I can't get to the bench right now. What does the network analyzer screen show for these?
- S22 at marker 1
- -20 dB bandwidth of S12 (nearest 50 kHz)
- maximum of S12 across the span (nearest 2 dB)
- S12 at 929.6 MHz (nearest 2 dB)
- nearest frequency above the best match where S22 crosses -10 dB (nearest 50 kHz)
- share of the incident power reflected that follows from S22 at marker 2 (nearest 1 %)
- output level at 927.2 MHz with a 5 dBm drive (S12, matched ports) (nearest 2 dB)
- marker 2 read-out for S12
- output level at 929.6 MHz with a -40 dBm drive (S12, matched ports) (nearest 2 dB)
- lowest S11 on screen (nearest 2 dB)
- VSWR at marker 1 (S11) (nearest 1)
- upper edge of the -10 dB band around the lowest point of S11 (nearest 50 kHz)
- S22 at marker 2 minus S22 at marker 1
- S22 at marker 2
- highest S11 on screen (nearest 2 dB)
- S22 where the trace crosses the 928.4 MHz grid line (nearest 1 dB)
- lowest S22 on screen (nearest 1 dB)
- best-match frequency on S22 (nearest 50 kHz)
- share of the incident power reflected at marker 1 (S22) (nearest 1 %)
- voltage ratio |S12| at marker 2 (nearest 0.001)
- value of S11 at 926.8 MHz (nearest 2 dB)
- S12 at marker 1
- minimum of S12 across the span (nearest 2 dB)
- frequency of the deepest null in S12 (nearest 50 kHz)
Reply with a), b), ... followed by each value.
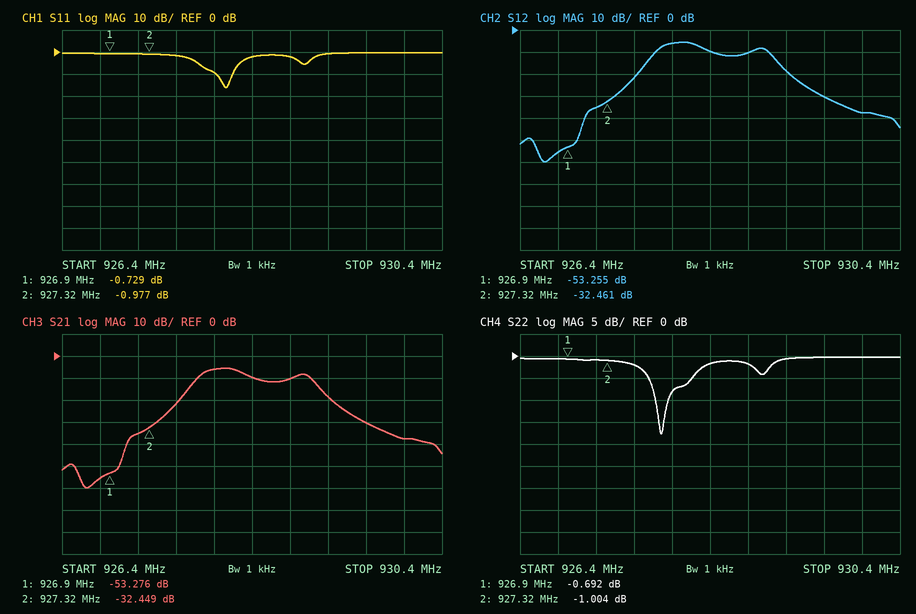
a) -0.692 dB
b) 1.90 MHz
c) -6 dB
d) -30 dB
e) 927.95 MHz
f) 79 %
g) -30 dBm
h) -32.461 dB
i) -70 dBm
j) -16 dB
k) 24
l) 928.20 MHz
m) -0.312 dB
n) -1.004 dB
o) 0 dB
p) -2 dB
q) -18 dB
r) 927.90 MHz
s) 85 %
t) 0.024
u) 0 dB
v) -53.255 dB
w) -60 dB
x) 926.65 MHz
